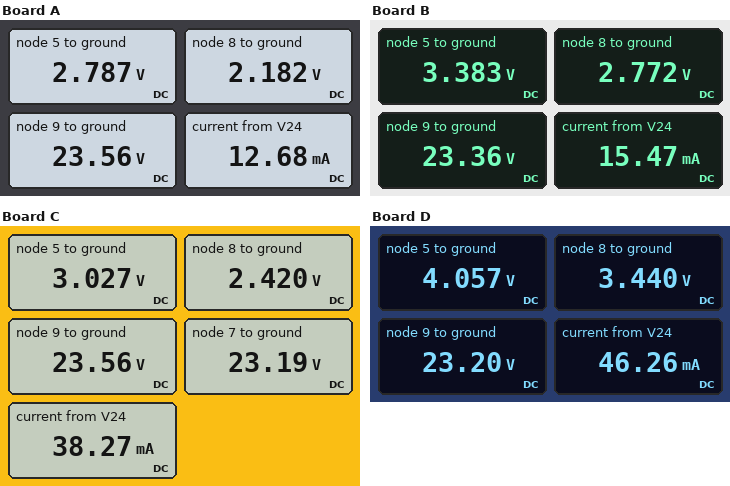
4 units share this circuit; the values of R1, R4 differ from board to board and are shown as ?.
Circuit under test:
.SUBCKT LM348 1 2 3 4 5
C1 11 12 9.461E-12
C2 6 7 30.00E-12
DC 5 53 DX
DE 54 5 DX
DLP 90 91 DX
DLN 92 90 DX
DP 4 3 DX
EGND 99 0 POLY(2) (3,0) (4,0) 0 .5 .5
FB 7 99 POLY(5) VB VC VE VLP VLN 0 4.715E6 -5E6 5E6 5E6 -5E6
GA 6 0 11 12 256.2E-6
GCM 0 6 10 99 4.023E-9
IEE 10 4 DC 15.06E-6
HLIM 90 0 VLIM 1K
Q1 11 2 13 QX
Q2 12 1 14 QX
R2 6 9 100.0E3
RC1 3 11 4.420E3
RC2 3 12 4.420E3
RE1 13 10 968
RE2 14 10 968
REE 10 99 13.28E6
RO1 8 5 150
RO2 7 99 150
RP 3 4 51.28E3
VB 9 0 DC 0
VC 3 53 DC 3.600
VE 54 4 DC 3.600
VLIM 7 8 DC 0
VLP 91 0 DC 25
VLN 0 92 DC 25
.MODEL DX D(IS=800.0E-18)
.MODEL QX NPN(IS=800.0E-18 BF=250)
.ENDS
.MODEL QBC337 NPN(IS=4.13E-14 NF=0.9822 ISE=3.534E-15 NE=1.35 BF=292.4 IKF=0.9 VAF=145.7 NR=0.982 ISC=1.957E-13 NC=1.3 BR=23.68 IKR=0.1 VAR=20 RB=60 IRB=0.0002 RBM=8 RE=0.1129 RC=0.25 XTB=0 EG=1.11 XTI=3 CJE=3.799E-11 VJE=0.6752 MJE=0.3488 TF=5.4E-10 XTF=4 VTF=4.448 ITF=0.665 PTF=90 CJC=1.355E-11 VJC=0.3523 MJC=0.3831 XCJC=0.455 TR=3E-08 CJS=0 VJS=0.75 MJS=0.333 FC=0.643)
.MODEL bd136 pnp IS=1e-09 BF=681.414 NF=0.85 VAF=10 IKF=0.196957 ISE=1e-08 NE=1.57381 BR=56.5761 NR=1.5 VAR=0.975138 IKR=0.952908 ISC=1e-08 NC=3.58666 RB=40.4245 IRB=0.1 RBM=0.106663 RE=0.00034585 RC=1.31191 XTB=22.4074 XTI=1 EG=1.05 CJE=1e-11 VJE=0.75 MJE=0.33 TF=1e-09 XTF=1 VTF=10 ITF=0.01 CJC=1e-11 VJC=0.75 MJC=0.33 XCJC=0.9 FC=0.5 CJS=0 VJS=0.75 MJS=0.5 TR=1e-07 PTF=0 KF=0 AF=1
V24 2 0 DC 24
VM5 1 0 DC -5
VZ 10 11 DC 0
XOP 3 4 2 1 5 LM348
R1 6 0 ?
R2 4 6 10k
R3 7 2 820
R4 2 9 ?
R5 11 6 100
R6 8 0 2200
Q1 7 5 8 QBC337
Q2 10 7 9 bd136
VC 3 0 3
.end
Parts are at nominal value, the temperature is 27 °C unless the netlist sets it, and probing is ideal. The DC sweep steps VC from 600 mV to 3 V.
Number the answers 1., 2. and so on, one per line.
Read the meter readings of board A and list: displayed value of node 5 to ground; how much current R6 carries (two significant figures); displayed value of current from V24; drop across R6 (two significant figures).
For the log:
1. 2.787 V
2. 990 µA
3. 12.68 mA
4. 2.2 V
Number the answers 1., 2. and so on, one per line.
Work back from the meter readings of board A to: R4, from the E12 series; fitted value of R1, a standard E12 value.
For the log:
1. 39 Ω
2. 270 Ω
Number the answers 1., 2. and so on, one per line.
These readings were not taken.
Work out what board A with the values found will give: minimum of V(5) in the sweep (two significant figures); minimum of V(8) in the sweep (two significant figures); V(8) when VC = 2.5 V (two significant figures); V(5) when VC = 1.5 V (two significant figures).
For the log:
1. 1.7 V
2. 1.1 V
3. 2.0 V
4. 2.1 V
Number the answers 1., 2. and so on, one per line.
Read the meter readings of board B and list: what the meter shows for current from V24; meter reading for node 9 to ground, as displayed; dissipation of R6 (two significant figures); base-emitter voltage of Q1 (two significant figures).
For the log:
1. 15.47 mA
2. 23.36 V
3. 3.5 mW
4. 610 mV
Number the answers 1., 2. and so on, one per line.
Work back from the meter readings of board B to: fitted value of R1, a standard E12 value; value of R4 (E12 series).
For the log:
1. 220 Ω
2. 47 Ω
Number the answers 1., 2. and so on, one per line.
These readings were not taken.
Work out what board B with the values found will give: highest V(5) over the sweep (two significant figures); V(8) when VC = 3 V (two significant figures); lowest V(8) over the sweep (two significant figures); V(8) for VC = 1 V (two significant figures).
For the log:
1. 3.4 V
2. 2.8 V
3. 1.2 V
4. 1.5 V
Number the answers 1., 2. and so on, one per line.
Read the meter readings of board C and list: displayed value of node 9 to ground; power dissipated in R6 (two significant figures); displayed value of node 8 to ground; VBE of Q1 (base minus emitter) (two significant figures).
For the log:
1. 23.56 V
2. 2.7 mW
3. 2.420 V
4. 610 mV
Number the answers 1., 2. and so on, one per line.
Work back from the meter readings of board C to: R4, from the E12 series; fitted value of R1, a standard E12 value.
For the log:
1. 12 Ω
2. 82 Ω
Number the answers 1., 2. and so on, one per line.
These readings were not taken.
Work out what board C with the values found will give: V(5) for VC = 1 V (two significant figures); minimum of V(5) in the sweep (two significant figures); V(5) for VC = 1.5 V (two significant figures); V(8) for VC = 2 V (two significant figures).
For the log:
1. 2.0 V
2. 1.8 V
3. 2.3 V
4. 1.9 V
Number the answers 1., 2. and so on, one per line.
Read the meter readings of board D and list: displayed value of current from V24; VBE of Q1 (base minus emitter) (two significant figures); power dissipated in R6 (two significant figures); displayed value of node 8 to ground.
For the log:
1. 46.26 mA
2. 620 mV
3. 5.4 mW
4. 3.440 V
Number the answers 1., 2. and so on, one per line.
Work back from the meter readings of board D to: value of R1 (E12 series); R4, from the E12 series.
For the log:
1. 68 Ω
2. 18 Ω
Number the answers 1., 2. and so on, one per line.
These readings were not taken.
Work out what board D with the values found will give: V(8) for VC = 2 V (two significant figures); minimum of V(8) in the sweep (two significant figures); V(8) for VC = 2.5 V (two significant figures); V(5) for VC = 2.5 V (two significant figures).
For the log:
1. 2.6 V
2. 1.4 V
3. 3.0 V
4. 3.6 V
